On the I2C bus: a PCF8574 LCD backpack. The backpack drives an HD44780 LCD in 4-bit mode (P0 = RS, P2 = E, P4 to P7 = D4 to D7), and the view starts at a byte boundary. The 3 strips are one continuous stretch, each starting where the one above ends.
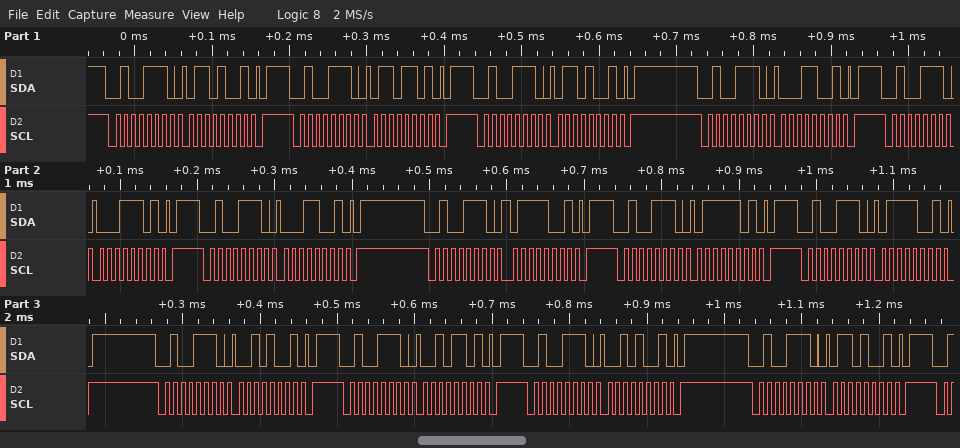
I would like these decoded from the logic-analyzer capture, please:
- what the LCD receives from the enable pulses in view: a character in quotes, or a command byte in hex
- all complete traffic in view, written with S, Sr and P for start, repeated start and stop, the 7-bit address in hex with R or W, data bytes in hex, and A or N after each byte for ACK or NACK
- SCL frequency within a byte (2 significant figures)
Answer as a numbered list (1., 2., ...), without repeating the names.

1. 'a' 'r'
2. S 27W A 69 A P S 27W A 6D A P S 27W A 69 A P S 27W A 19 A P S 27W A 1D A P S 27W A 19 A P S 27W A 79 A P S 27W A 7D A P S 27W A 79 A P S 27W A 29 A P S 27W A 2D A P S 27W A 29 A P S 27W A 69 A P
3. 100 kHz
